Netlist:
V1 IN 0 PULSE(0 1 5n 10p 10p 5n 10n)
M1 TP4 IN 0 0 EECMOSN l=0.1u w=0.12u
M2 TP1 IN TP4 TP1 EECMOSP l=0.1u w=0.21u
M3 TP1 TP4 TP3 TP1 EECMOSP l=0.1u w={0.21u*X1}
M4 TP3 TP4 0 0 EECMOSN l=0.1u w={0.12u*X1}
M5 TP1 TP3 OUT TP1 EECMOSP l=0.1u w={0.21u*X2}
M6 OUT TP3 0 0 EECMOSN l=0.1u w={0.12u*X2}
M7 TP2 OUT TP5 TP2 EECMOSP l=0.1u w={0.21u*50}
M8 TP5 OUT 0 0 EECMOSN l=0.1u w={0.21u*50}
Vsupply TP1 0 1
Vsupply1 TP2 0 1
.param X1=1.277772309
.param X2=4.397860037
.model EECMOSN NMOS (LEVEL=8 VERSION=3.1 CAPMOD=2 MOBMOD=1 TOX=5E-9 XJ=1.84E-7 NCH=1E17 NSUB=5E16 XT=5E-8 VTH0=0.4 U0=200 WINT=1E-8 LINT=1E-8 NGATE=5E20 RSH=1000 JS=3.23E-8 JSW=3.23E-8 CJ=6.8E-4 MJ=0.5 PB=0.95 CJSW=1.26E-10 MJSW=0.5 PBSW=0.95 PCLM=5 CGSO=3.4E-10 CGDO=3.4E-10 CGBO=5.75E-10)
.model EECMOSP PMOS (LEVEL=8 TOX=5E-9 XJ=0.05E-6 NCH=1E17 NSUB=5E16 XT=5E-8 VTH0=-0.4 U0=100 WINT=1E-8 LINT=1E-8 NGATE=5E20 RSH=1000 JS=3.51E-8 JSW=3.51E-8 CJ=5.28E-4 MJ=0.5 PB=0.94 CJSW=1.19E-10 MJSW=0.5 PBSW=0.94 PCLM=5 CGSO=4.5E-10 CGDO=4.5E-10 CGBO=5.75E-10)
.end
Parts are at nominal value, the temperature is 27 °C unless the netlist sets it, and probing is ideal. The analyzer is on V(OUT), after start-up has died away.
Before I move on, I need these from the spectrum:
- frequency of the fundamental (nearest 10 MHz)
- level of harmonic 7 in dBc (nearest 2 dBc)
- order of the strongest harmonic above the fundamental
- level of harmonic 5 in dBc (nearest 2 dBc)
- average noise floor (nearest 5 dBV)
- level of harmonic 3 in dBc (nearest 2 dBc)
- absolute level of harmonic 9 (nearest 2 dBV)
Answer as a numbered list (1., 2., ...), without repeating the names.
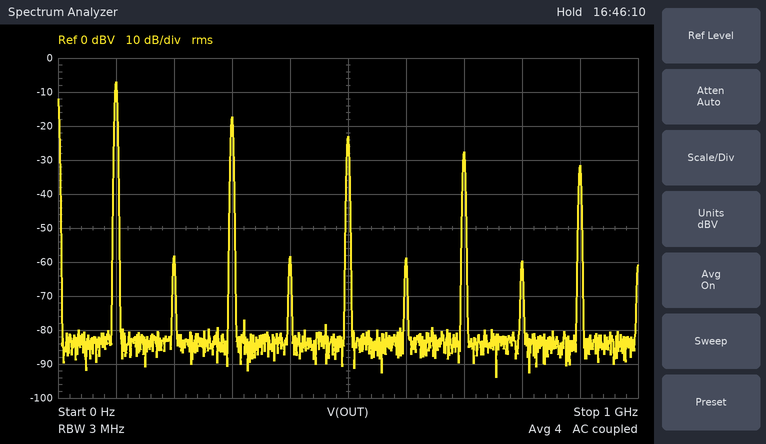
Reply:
1. 100 MHz
2. -20 dBc
3. 3
4. -16 dBc
5. -85 dBV
6. -10 dBc
7. -32 dBV
